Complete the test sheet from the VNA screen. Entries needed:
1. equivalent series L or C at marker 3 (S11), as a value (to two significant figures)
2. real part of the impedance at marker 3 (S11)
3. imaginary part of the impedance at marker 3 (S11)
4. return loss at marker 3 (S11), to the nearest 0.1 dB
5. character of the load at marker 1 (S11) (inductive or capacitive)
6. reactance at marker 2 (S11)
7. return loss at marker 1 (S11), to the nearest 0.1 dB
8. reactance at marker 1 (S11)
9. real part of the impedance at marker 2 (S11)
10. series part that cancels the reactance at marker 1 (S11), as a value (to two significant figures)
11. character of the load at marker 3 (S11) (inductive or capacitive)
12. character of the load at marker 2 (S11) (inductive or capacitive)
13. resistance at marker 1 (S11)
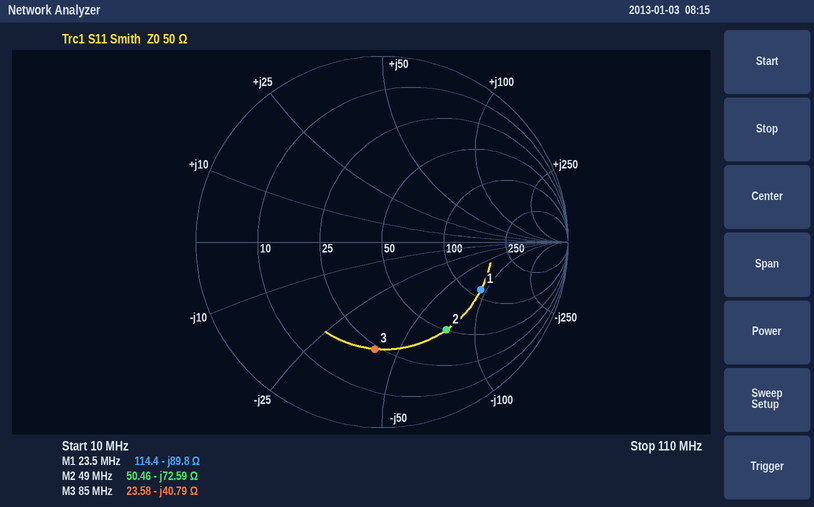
46 pF
23.58 Ω
-40.79 Ω
4.8 dB
capacitive
-72.59 Ω
4.6 dB
-89.8 Ω
50.46 Ω
610 nH
capacitive
capacitive
114.4 Ω
